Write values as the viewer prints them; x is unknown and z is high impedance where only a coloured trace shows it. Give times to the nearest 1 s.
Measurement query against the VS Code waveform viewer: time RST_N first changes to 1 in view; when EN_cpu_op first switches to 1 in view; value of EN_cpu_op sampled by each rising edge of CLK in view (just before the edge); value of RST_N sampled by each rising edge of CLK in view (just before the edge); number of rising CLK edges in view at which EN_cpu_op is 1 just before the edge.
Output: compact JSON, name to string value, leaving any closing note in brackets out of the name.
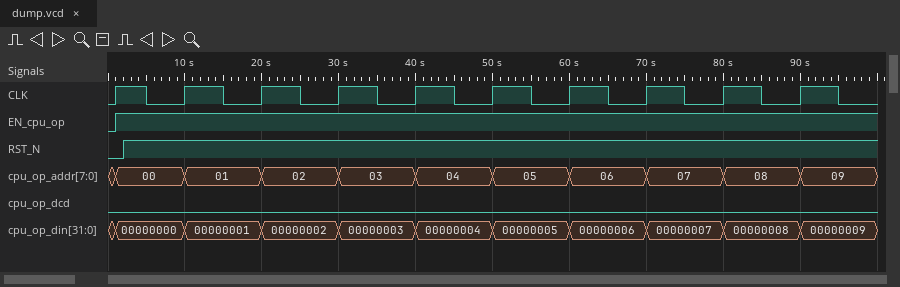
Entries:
{"time RST_N first changes to 1 in view": "2 s", "when EN_cpu_op first switches to 1 in view": "1 s", "value of EN_cpu_op sampled by each rising edge of CLK in view": "0 1 1 1 1 1 1 1 1 1", "value of RST_N sampled by each rising edge of CLK in view": "0 1 1 1 1 1 1 1 1 1", "number of rising CLK edges in view at which EN_cpu_op is 1 just before the edge": "9"}
